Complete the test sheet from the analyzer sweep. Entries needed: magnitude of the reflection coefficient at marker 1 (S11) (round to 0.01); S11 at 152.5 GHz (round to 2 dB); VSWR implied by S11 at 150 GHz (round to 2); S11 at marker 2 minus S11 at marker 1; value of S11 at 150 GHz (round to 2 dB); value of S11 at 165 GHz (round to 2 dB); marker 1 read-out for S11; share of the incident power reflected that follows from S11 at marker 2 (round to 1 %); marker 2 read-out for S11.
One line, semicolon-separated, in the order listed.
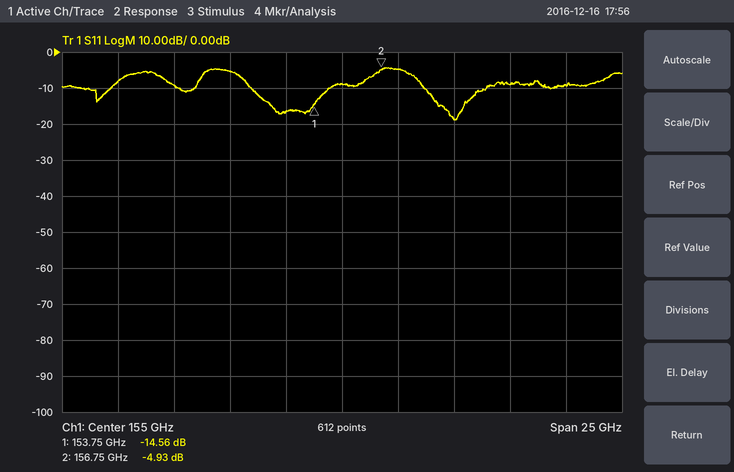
0.19; -16 dB; 4; 9.63 dB; -6 dB; -10 dB; -14.56 dB; 32 %; -4.93 dB
